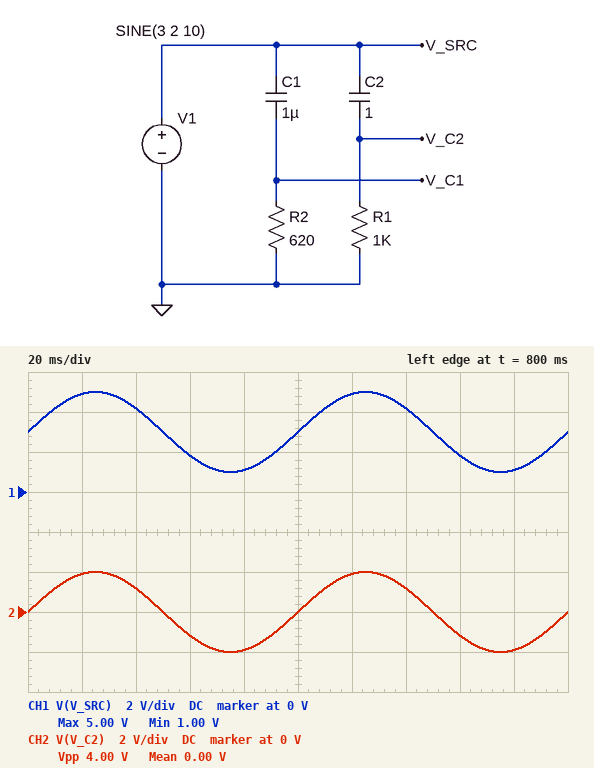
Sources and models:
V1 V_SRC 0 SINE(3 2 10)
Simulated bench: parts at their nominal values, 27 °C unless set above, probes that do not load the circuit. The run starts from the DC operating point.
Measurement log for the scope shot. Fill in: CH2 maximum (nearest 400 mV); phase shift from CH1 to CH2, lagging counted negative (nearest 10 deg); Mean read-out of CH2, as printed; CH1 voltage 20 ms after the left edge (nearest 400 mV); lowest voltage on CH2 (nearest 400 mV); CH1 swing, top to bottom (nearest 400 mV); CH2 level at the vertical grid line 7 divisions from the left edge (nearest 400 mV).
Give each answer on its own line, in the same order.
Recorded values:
2.0 V
0 deg
0.00 V
4.8 V
-2.0 V
4.0 V
1.2 V
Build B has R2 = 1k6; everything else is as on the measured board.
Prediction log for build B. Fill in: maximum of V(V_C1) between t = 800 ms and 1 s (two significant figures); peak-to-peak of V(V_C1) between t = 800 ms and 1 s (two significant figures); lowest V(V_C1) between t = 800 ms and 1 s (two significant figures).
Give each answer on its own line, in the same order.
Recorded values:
200 mV
400 mV
-200 mV
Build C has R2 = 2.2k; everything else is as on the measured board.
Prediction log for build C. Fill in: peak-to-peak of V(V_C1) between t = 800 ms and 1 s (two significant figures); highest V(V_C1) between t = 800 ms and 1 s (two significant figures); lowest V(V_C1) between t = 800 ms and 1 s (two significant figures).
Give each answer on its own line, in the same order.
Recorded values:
550 mV
270 mV
-270 mV
